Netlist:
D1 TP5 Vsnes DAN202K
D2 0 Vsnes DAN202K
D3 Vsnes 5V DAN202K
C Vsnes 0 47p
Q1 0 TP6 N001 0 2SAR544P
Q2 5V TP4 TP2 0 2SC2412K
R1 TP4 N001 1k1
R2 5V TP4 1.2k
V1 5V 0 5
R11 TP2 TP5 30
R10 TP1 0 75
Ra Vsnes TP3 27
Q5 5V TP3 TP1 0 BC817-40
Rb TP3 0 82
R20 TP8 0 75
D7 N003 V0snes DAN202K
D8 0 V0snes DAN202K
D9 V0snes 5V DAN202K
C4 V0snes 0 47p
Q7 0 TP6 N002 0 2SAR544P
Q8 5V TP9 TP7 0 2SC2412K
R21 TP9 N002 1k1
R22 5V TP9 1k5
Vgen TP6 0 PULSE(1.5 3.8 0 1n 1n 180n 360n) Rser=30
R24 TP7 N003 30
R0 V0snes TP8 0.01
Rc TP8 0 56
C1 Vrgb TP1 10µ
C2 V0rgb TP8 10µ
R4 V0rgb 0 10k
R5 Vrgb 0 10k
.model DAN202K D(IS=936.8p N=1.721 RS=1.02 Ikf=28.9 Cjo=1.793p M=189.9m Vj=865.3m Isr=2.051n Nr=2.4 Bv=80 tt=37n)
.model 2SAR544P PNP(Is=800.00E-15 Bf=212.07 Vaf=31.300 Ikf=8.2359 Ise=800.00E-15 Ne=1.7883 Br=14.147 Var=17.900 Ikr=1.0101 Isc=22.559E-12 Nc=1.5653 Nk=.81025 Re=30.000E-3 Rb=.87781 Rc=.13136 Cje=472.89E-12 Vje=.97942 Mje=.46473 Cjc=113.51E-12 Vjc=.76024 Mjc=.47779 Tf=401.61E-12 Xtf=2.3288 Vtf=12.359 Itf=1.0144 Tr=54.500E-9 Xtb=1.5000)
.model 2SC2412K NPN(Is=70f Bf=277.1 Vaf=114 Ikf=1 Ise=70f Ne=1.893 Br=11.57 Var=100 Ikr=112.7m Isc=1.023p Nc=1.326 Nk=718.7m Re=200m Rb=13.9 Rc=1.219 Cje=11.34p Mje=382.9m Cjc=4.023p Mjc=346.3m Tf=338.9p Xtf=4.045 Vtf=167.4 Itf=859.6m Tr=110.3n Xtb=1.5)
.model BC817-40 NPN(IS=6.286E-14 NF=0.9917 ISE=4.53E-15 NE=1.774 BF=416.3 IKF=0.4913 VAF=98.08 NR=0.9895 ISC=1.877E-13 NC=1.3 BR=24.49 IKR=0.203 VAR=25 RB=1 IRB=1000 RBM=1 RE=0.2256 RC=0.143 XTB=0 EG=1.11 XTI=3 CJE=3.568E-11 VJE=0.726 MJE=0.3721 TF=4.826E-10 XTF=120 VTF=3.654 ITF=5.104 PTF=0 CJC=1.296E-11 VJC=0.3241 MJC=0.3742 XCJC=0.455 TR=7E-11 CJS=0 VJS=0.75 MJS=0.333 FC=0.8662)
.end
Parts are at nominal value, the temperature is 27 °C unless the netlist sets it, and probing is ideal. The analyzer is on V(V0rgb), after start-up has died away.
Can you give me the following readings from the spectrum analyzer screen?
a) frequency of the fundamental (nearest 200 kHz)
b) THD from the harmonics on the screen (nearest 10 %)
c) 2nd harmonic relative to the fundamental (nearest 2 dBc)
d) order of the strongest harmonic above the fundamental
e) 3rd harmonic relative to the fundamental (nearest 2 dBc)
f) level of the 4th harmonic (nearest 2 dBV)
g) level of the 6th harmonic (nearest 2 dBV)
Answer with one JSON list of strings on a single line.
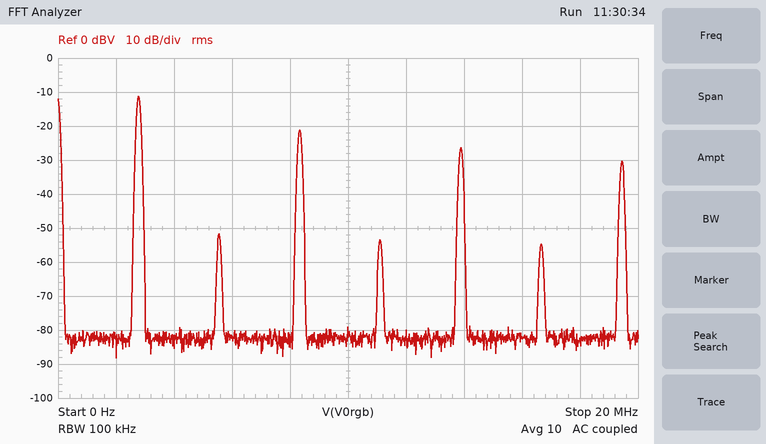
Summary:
["2.8 MHz", "40 %", "-40 dBc", "3", "-10 dBc", "-54 dBV", "-54 dBV"]
